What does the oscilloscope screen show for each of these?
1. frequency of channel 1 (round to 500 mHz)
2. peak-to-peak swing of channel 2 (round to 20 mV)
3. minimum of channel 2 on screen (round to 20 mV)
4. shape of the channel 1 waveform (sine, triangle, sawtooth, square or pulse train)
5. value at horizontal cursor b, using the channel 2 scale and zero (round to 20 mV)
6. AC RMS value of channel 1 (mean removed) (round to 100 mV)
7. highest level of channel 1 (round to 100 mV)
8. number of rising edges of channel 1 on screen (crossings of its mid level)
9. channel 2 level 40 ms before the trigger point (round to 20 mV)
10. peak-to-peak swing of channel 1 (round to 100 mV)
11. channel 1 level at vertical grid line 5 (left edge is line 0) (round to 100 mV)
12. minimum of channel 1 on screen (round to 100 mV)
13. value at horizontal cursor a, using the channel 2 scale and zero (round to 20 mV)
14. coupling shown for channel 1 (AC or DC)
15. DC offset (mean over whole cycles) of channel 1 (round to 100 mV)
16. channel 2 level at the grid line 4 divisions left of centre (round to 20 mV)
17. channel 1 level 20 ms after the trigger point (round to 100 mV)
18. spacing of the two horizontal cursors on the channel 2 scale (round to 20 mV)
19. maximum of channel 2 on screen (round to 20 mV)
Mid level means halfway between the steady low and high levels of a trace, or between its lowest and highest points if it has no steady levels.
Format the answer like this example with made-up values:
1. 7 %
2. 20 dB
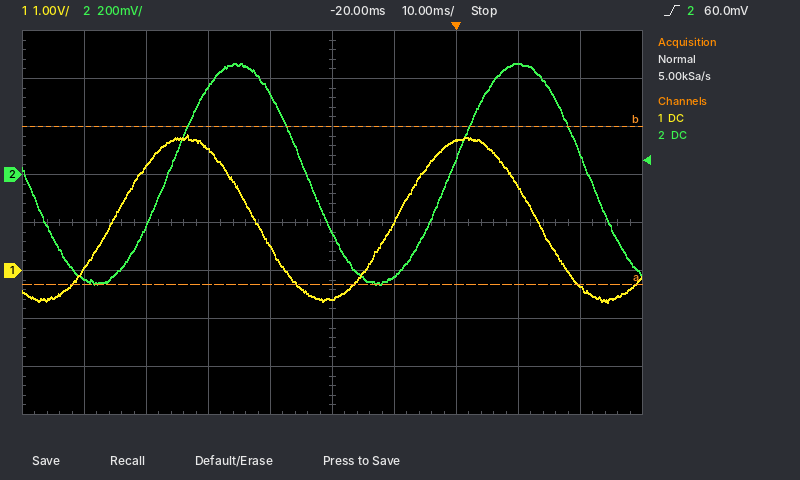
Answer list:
1. 22.0 Hz
2. 920 mV
3. -460 mV
4. sine
5. 200 mV
6. 1.2 V
7. 2.8 V
8. 2
9. 360 mV
10. 3.5 V
11. -600 mV
12. -700 mV
13. -460 mV
14. DC
15. 1.1 V
16. -440 mV
17. -300 mV
18. 660 mV
19. 460 mV
